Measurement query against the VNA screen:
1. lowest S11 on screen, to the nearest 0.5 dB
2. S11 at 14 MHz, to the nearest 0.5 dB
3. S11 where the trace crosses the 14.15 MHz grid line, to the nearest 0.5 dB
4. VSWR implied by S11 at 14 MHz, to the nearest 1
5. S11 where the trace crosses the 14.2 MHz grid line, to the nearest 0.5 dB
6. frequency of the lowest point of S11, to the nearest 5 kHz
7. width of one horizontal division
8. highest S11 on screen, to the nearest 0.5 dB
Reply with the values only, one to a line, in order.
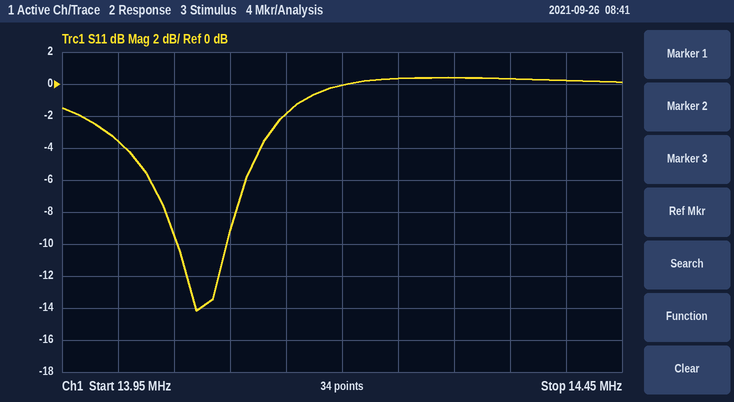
-14.0 dB
-3.5 dB
-2.0 dB
5
0.0 dB
14.070 MHz
50 kHz
0.5 dB
